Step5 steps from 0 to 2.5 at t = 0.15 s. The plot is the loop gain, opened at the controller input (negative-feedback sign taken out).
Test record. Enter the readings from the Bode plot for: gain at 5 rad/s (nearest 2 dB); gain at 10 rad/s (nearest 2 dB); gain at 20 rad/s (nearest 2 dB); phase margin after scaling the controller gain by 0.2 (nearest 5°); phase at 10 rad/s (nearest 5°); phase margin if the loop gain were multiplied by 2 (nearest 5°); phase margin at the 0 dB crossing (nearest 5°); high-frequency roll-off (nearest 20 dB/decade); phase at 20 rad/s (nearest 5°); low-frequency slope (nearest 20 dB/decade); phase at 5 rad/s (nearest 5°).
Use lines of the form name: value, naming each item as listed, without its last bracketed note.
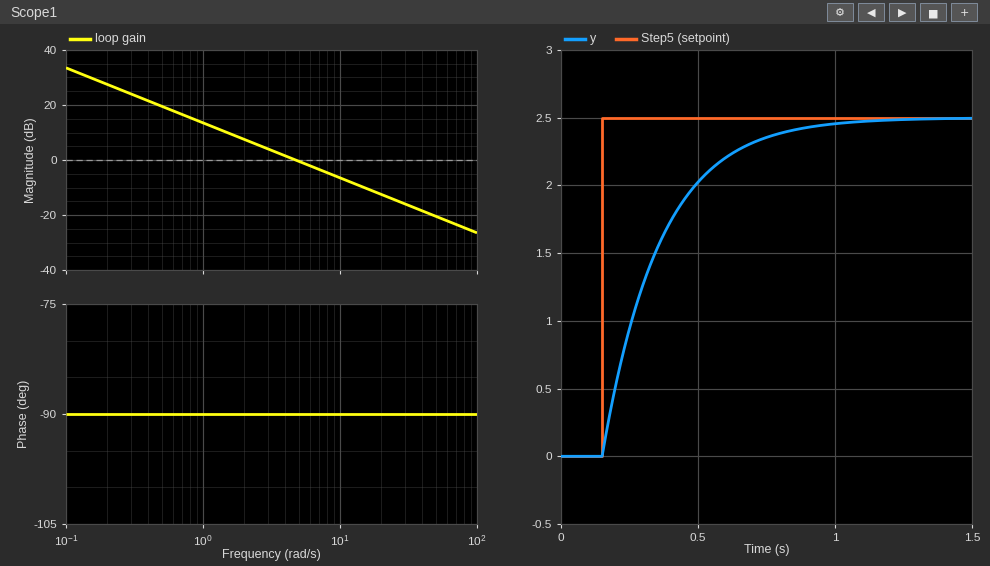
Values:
gain at 5 rad/s: 0 dB
gain at 10 rad/s: -6 dB
gain at 20 rad/s: -12 dB
phase margin after scaling the controller gain by 0.2: 90°
phase at 10 rad/s: -90°
phase margin if the loop gain were multiplied by 2: 90°
phase margin at the 0 dB crossing: 90°
high-frequency roll-off: -20 dB/decade
phase at 20 rad/s: -90°
low-frequency slope: -20 dB/decade
phase at 5 rad/s: -90°
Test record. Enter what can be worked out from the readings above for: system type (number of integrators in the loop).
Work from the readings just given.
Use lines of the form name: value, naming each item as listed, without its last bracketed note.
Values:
system type: 1
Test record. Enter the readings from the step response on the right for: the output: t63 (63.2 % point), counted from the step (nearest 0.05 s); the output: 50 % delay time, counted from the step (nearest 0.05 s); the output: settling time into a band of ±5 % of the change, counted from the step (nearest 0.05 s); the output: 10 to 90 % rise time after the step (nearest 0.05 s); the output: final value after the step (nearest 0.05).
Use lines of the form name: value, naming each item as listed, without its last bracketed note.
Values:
the output: t63 (63.2 % point), counted from the step: 0.20 s
the output: 50 % delay time, counted from the step: 0.15 s
the output: settling time into a band of ±5 % of the change, counted from the step: 0.65 s
the output: 10 to 90 % rise time after the step: 0.45 s
the output: final value after the step: 2.50
